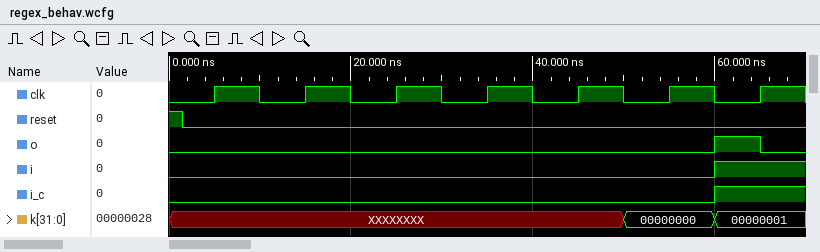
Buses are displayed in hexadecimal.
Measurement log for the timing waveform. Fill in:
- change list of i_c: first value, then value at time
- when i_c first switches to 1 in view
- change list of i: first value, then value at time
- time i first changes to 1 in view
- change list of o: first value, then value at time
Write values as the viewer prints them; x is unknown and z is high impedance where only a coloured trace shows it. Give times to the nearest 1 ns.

0, 1 at 60 ns
60 ns
0, 1 at 60 ns
60 ns
0, 1 at 60 ns, 0 at 65 ns
